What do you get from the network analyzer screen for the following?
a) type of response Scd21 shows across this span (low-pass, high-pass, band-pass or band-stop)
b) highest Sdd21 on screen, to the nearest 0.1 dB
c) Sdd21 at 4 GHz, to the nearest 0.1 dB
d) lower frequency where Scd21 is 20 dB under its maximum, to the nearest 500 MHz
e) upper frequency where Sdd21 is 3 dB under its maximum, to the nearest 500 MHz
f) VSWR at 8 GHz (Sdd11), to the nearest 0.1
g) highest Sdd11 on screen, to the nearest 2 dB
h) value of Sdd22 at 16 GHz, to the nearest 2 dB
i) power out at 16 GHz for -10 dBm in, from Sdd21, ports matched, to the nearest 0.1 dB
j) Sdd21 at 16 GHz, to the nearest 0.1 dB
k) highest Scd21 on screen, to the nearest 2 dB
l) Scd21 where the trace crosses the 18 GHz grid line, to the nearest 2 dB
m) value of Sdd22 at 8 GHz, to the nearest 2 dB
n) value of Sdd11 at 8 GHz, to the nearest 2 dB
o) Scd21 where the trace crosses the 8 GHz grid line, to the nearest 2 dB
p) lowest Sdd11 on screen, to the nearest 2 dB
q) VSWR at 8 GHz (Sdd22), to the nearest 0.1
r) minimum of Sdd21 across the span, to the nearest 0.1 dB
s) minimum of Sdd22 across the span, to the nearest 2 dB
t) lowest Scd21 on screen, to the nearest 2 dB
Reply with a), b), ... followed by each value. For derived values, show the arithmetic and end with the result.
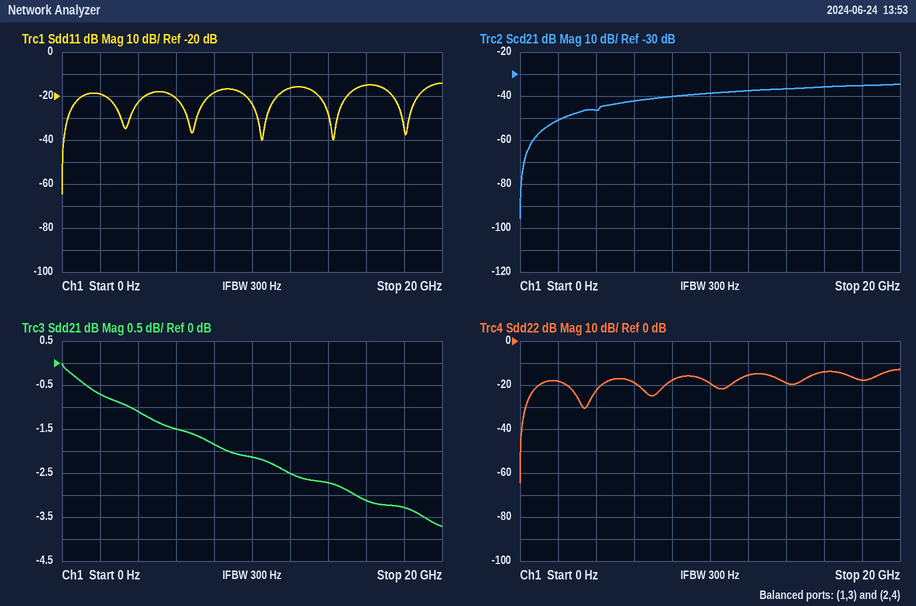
a) high-pass
b) 0.0 dB
c) -1.1 dB
d) 1.5 GHz
e) 15.5 GHz
f) |Γ| = 10^(-18/20) = 0.1259; VSWR = (1 + 0.1259)/(1 − 0.1259) ≈ 1.3
g) -14 dB
h) -14 dB
i) -10 dBm + (-3.1 dB) = -13.1 dBm
j) -3.1 dB
k) -34 dB
l) -36 dB
m) -18 dB
n) -18 dB
o) -40 dB
p) -64 dB
q) |Γ| = 10^(-18/20) = 0.1259; VSWR = (1 + 0.1259)/(1 − 0.1259) ≈ 1.3
r) -3.7 dB
s) -64 dB
t) -96 dB
